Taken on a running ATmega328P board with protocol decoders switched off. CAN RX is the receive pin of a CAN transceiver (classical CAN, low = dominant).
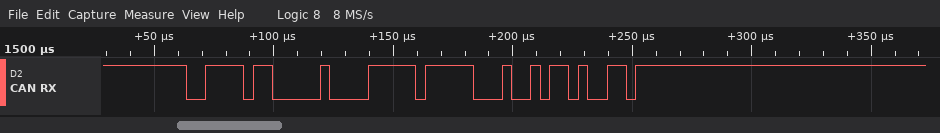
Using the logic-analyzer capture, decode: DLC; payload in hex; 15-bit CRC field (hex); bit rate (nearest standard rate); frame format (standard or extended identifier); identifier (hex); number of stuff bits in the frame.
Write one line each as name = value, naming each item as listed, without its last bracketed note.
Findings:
DLC = 1
payload in hex = FF
15-bit CRC field = 0x4969
bit rate = 250 kbit/s
frame format = standard
identifier = 0x3D8
number of stuff bits in the frame = 3
